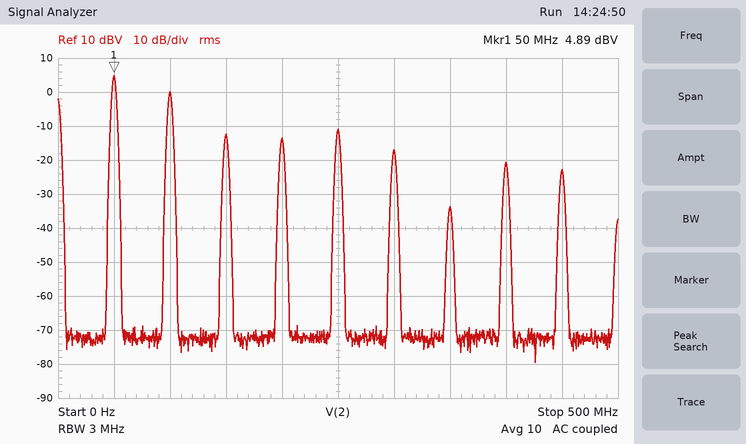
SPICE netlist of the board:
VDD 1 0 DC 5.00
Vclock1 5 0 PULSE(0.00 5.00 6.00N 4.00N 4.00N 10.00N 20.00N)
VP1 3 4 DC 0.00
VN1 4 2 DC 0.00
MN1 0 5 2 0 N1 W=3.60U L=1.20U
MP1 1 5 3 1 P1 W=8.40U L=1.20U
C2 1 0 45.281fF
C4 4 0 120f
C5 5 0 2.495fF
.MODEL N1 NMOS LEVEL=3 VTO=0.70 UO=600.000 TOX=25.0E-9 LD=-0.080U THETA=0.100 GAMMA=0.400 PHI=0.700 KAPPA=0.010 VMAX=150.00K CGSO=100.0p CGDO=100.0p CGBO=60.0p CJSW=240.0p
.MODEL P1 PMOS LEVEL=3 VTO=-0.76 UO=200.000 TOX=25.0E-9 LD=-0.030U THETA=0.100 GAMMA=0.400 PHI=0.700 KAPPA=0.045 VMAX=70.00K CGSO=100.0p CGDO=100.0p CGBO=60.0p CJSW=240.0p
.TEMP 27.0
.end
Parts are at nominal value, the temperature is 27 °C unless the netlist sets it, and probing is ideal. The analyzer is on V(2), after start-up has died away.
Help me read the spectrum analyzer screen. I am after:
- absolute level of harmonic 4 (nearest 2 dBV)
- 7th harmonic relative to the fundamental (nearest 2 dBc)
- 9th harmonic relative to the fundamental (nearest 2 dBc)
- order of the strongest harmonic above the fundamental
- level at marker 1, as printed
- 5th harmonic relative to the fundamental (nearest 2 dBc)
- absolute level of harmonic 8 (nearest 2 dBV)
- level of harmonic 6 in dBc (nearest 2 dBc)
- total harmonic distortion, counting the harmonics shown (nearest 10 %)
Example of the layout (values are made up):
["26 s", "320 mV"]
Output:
["-14 dBV", "-38 dBc", "-28 dBc", "2", "4.89 dBV", "-16 dBc", "-20 dBV", "-22 dBc", "60 %"]
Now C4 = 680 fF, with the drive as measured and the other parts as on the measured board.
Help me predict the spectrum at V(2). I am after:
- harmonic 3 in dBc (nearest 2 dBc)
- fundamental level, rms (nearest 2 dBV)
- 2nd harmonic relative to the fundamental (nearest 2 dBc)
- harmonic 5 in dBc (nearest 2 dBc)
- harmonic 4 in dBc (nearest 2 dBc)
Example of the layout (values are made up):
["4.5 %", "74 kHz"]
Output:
["-22 dBc", "2 dBV", "-8 dBc", "-38 dBc", "-36 dBc"]
